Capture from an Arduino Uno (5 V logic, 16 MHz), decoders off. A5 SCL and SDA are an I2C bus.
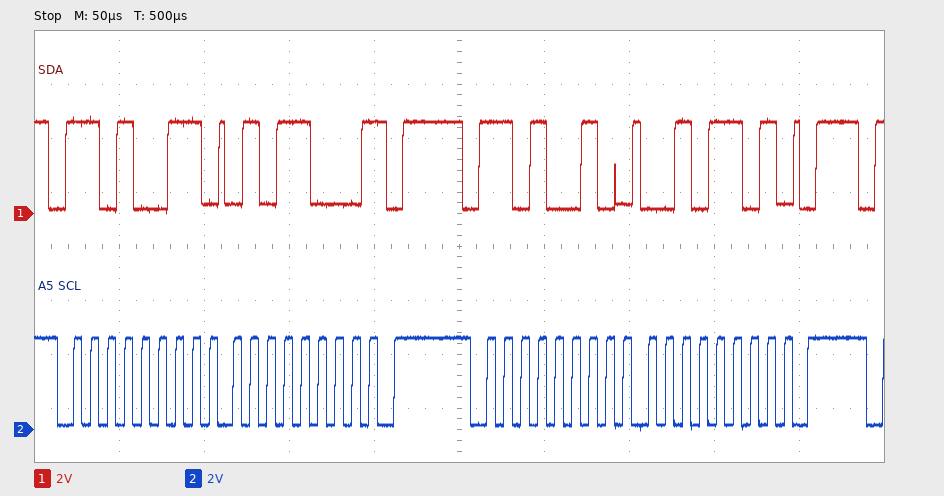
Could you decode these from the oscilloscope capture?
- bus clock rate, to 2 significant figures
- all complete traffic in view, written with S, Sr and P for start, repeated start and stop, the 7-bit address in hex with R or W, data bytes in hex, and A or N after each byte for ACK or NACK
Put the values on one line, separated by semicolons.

100 kHz; S 69R A 58 N P S 69W A 2D A P
